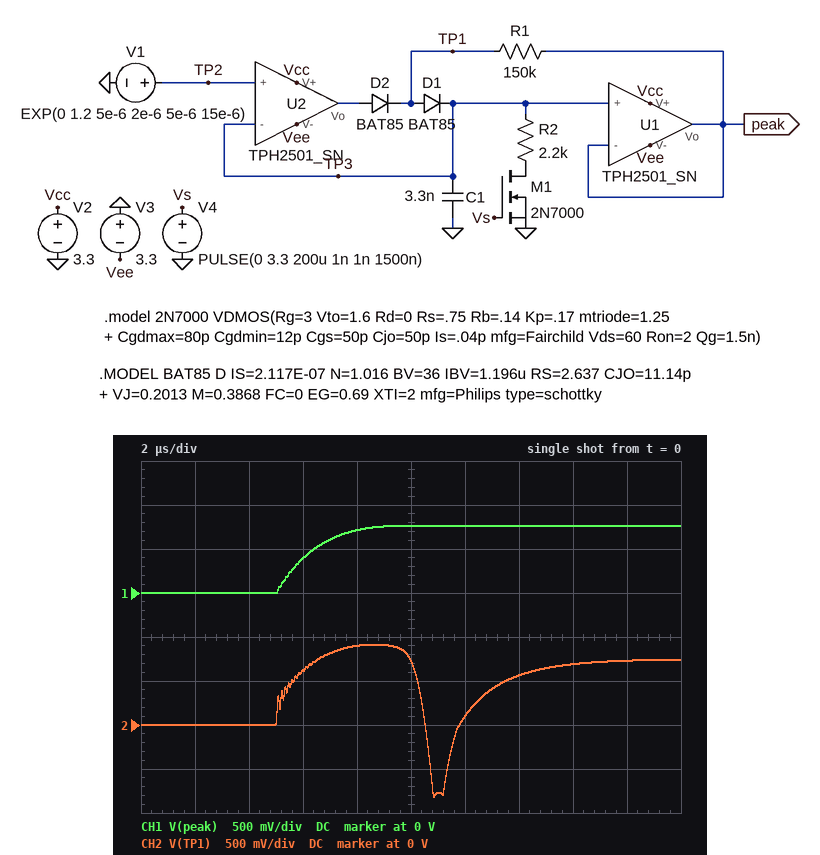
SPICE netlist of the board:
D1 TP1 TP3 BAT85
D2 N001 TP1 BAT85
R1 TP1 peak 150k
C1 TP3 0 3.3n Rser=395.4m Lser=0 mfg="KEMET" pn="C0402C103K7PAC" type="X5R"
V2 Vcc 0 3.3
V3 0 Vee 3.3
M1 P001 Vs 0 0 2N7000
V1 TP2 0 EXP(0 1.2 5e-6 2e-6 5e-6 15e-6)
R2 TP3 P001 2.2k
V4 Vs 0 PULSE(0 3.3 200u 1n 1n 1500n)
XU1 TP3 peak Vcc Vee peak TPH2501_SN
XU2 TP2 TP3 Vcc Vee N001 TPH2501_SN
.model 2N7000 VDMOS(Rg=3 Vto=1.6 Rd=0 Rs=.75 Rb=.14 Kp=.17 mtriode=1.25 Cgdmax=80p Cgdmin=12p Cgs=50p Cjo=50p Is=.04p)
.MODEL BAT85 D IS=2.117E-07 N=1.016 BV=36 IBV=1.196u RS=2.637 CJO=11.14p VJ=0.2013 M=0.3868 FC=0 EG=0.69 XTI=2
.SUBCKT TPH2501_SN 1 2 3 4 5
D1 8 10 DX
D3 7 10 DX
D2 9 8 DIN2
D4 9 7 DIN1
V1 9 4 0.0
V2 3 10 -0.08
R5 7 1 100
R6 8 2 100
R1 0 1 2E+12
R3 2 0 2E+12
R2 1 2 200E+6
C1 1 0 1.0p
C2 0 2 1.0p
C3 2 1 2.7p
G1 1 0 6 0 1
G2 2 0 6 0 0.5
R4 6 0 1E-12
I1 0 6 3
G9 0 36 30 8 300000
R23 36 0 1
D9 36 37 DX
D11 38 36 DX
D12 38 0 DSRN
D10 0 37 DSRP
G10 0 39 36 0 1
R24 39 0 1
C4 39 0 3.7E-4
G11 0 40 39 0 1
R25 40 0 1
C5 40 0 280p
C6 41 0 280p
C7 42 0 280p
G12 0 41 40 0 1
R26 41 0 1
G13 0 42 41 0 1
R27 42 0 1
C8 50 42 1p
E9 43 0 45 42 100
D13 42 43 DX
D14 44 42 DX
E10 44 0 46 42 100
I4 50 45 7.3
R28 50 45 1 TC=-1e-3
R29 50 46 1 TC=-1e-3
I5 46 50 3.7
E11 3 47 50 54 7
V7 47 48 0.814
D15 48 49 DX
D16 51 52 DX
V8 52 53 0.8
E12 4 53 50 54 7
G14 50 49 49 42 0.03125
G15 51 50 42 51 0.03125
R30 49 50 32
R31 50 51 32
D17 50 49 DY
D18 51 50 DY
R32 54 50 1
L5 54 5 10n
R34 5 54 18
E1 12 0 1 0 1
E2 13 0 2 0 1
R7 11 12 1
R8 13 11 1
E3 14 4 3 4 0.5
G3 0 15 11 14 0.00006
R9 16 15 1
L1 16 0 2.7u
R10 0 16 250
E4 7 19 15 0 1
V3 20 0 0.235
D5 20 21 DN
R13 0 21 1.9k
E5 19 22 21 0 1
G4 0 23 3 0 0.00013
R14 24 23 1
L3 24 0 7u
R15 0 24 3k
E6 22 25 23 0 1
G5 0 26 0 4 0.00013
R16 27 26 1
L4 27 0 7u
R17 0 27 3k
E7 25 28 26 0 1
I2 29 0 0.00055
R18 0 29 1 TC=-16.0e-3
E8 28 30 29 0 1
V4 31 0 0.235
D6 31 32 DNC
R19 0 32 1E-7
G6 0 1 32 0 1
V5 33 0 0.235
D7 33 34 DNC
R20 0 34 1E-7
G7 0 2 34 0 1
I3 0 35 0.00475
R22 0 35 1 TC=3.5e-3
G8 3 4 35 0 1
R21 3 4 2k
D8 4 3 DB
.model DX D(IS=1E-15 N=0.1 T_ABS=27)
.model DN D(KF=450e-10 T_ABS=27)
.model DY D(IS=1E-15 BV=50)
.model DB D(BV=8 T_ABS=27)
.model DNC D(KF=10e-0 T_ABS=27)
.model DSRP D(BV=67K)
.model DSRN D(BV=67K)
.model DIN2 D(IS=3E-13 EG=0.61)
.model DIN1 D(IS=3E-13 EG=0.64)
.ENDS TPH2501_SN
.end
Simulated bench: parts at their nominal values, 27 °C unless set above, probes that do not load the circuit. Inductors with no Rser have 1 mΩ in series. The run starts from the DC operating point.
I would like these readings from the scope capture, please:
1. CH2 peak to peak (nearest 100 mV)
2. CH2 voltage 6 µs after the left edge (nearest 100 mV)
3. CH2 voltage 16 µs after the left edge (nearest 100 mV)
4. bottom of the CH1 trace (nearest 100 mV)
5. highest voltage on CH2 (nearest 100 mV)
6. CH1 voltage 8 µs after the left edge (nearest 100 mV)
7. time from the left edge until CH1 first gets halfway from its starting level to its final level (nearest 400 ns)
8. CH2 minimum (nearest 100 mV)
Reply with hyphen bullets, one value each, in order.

- 1.7 V
- 600 mV
- 700 mV
- 0 V
- 900 mV
- 700 mV
- 6.0 µs
- -800 mV
